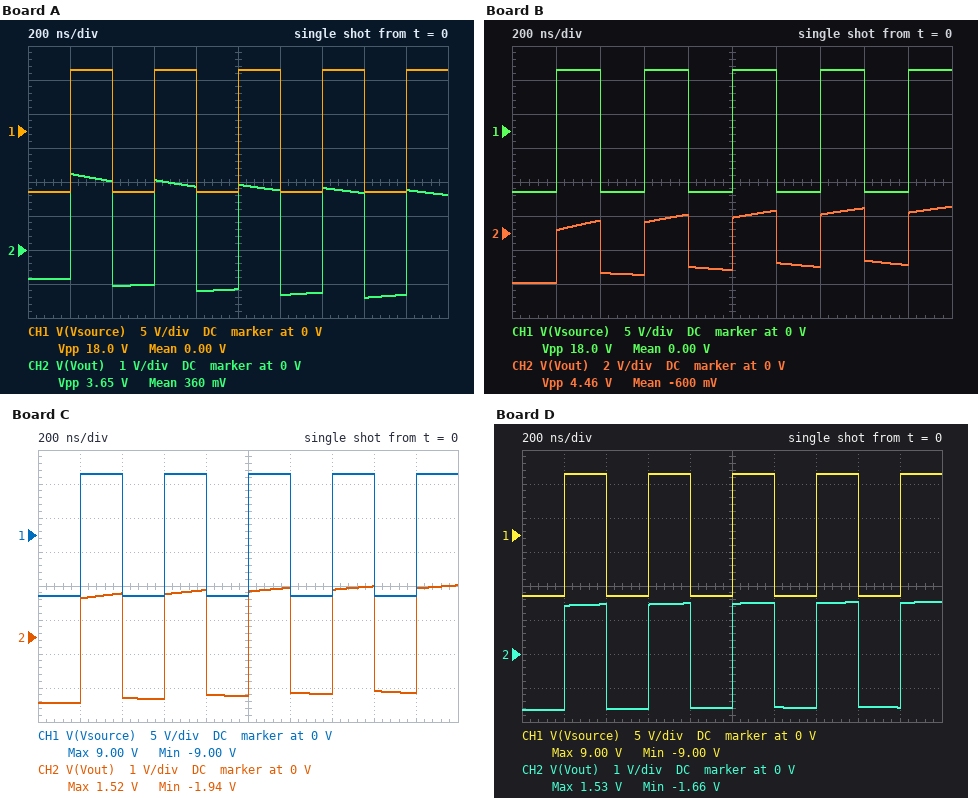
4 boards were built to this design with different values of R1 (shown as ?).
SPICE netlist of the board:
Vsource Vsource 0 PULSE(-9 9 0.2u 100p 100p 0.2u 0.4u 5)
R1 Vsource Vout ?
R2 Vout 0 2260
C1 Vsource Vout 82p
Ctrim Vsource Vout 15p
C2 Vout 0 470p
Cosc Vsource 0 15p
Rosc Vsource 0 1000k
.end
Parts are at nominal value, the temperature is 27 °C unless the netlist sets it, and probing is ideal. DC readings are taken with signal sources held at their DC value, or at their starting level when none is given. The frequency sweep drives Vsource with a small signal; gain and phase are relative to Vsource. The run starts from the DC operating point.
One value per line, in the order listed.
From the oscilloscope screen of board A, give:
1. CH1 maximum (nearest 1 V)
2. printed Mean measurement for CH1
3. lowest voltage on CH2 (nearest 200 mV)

9 V
0.00 V
-1.4 V
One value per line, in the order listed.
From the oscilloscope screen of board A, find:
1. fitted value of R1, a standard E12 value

22 kΩ
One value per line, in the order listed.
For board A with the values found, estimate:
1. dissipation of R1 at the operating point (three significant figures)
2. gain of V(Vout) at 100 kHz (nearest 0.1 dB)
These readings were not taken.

3.03 mW
-18.0 dB
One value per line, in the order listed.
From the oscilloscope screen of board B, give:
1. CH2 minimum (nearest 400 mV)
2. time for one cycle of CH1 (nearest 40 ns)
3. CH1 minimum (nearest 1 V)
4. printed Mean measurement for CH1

-2.8 V
400 ns
-9 V
0.00 V
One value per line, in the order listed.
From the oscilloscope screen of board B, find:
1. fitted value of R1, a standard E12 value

4.7 kΩ
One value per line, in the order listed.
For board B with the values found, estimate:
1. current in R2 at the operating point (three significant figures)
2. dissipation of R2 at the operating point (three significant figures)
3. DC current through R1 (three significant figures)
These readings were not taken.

1.29 mA
3.78 mW
1.29 mA
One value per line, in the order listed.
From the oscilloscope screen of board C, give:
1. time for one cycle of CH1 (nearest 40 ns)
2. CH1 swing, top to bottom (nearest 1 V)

400 ns
18 V
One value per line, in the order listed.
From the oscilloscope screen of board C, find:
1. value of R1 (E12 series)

8.2 kΩ
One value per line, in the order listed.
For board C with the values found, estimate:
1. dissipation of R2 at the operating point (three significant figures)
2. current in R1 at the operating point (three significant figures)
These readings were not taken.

1.67 mW
860 µA
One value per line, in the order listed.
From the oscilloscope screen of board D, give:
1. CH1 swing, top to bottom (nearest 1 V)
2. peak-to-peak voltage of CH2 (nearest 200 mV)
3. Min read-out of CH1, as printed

18 V
3.2 V
-9.00 V
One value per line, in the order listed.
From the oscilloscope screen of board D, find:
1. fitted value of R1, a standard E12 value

10 kΩ
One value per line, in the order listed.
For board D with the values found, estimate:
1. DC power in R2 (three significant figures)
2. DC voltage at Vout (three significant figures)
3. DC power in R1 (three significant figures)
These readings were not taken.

1.22 mW
-1.66 V
5.39 mW
